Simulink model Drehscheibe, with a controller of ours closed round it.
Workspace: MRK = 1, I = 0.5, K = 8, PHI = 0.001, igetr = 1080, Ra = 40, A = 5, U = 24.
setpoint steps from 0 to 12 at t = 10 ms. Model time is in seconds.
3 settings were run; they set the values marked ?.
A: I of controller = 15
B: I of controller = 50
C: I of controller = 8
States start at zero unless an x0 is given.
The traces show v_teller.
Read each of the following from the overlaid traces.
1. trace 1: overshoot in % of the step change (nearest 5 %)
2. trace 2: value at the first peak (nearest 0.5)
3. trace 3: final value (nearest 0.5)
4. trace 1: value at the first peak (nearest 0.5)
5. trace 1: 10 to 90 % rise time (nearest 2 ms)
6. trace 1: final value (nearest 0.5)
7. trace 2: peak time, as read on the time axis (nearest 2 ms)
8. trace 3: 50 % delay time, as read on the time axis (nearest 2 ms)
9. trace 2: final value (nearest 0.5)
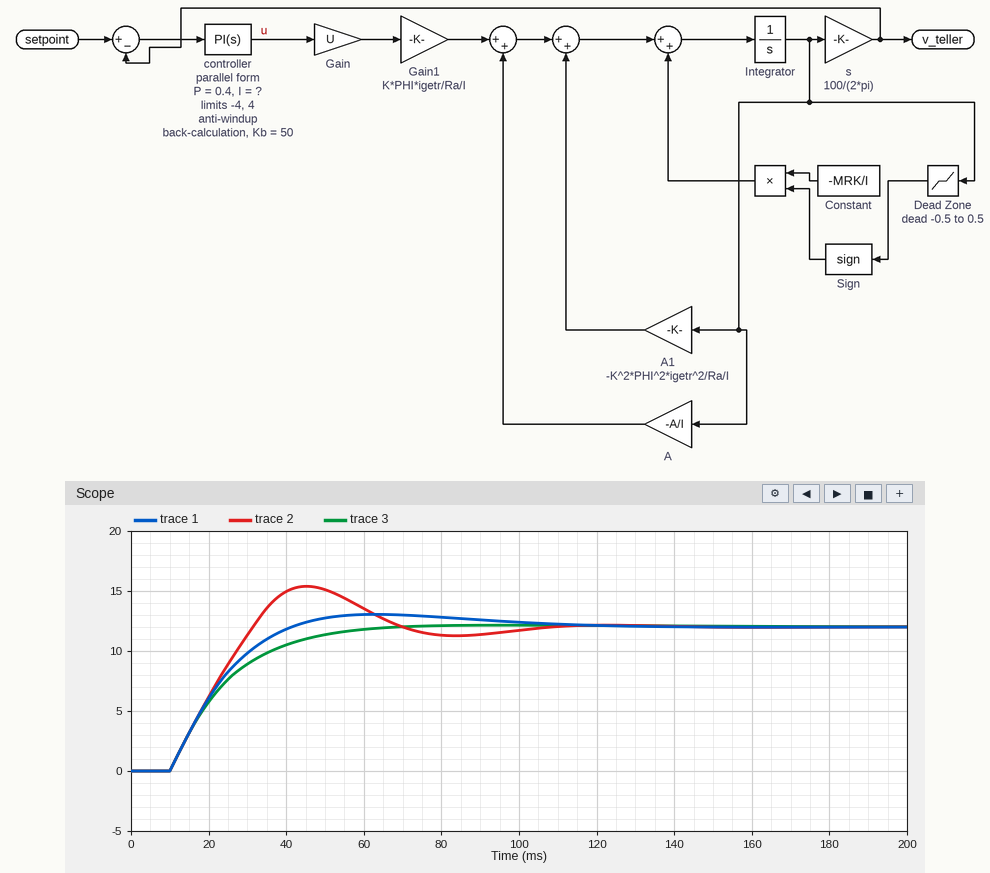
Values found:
10 %
15.5
12.0
13.0
22 ms
12.0
46 ms
20 ms
12.0
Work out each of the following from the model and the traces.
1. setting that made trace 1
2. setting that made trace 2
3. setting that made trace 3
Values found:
A
B
C
